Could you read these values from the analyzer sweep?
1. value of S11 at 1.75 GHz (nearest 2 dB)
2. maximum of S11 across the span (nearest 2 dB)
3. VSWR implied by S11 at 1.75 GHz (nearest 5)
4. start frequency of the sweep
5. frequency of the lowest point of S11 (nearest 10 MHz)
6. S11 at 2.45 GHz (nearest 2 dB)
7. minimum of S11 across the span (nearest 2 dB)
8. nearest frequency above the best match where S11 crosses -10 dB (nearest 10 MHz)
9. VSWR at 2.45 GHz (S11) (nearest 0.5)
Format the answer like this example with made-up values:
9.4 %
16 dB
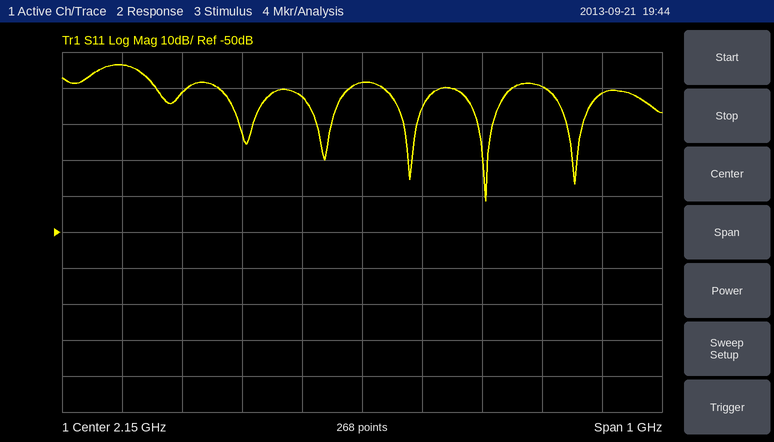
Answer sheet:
-4 dB
-4 dB
5
1.65 GHz
2.36 GHz
-10 dB
-42 dB
2.40 GHz
2.0
